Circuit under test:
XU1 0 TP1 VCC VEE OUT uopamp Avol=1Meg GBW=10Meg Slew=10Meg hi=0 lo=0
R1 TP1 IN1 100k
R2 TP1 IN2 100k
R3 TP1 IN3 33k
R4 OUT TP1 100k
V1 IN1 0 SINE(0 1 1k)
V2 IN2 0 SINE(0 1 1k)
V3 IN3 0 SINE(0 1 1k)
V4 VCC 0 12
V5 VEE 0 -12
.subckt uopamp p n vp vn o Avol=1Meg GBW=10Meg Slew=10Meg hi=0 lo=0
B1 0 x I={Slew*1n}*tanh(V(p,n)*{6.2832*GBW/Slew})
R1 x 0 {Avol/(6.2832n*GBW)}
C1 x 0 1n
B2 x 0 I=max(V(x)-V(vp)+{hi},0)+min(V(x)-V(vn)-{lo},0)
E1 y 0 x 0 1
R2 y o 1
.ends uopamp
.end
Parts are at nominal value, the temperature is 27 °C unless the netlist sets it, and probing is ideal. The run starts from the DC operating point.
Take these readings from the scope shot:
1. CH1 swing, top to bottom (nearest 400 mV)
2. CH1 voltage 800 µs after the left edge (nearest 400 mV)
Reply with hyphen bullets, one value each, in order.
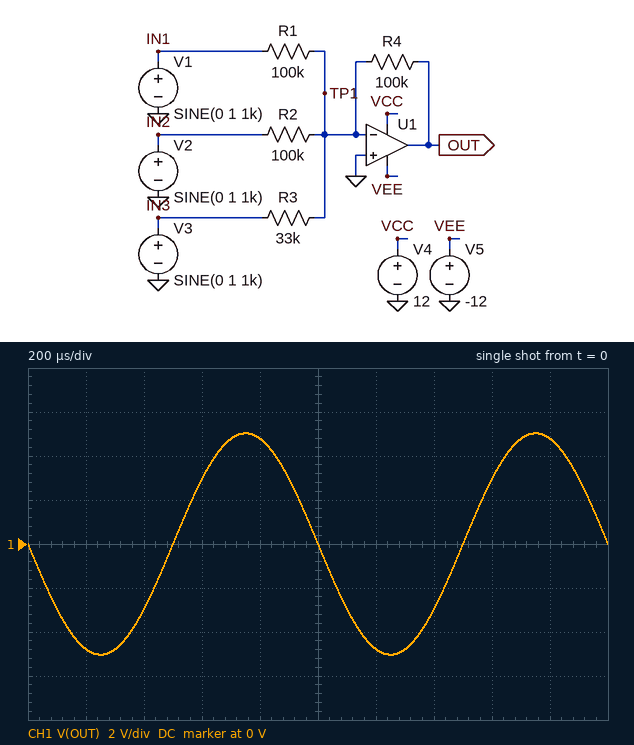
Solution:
- 10.0 V
- 4.8 V
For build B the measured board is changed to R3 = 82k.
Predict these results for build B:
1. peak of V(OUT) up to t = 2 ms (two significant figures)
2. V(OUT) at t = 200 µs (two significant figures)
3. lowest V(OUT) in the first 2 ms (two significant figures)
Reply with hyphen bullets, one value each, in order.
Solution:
- 3.2 V
- -3.1 V
- -3.2 V
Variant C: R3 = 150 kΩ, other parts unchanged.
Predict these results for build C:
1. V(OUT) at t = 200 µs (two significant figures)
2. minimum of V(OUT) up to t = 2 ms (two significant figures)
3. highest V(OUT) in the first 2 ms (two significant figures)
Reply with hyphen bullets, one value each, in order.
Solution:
- -2.5 V
- -2.7 V
- 2.7 V
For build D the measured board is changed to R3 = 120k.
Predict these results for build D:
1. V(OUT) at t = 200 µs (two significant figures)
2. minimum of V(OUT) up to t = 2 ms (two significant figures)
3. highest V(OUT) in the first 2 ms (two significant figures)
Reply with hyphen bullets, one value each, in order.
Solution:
- -2.7 V
- -2.8 V
- 2.8 V
